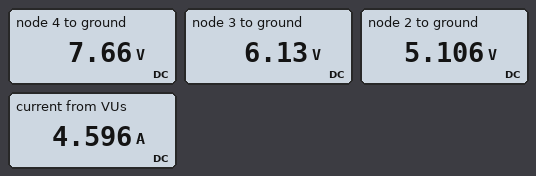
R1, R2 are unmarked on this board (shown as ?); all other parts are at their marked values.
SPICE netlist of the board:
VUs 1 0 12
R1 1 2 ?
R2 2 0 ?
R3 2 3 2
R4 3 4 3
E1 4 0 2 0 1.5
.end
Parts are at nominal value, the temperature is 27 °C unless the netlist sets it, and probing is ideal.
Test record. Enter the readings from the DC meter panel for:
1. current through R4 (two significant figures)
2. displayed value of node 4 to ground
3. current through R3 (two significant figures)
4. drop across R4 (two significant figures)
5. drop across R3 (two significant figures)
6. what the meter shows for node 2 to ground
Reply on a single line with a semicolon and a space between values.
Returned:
510 mA; 7.66 V; 510 mA; 1.5 V; 1.0 V; 5.106 V
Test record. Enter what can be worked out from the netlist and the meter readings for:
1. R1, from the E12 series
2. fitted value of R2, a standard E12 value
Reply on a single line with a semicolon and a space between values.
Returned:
1.5 Ω; 1 Ω
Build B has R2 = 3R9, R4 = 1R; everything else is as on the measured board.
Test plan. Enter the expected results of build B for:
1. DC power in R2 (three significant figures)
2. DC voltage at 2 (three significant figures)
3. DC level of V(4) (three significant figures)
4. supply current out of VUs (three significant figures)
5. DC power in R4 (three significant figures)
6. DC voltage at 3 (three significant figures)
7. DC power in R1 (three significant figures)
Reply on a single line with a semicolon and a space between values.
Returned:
28.7 W; 10.6 V; 15.9 V; 949 mA; 3.11 W; 14.1 V; 1.35 W
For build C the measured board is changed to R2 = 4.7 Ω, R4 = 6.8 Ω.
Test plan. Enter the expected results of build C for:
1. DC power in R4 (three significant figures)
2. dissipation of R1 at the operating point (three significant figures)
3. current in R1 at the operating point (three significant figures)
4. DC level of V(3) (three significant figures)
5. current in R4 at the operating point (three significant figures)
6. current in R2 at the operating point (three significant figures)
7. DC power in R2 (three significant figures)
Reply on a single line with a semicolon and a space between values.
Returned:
2.08 W; 3.45 W; 1.52 A; 10.8 V; 553 mA; 2.07 A; 20.1 W
